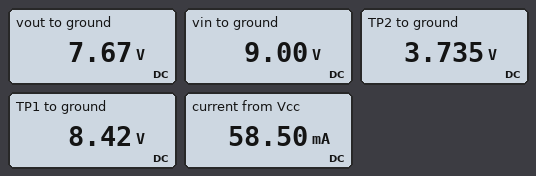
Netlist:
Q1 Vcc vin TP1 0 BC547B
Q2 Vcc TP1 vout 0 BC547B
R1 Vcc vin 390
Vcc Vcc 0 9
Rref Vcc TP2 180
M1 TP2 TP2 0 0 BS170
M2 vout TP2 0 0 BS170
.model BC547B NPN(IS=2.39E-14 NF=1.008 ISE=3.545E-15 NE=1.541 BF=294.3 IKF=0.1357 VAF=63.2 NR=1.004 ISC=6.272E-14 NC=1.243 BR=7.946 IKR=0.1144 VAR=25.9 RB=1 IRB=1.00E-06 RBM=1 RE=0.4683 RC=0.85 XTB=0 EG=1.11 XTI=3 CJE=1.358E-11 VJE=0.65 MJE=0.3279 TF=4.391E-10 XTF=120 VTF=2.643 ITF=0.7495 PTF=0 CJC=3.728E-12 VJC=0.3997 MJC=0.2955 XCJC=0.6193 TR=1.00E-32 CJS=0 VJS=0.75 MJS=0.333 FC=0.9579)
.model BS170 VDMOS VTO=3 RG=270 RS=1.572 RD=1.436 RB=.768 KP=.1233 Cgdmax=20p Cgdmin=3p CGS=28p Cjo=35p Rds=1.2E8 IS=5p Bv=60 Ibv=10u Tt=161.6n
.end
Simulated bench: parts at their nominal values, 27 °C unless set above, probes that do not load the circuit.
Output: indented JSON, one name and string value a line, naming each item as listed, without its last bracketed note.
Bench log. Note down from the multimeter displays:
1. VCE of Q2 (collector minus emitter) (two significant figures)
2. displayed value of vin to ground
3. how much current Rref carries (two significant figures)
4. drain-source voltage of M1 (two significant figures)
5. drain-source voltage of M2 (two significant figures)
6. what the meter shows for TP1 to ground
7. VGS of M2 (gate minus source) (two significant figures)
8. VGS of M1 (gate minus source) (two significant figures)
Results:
{
  "VCE of Q2 (collector minus emitter)": "1.3 V",
  "displayed value of vin to ground": "9.00 V",
  "how much current Rref carries": "29 mA",
  "drain-source voltage of M1": "3.7 V",
  "drain-source voltage of M2": "7.7 V",
  "what the meter shows for TP1 to ground": "8.42 V",
  "VGS of M2 (gate minus source)": "3.7 V",
  "VGS of M1 (gate minus source)": "3.7 V"
}
